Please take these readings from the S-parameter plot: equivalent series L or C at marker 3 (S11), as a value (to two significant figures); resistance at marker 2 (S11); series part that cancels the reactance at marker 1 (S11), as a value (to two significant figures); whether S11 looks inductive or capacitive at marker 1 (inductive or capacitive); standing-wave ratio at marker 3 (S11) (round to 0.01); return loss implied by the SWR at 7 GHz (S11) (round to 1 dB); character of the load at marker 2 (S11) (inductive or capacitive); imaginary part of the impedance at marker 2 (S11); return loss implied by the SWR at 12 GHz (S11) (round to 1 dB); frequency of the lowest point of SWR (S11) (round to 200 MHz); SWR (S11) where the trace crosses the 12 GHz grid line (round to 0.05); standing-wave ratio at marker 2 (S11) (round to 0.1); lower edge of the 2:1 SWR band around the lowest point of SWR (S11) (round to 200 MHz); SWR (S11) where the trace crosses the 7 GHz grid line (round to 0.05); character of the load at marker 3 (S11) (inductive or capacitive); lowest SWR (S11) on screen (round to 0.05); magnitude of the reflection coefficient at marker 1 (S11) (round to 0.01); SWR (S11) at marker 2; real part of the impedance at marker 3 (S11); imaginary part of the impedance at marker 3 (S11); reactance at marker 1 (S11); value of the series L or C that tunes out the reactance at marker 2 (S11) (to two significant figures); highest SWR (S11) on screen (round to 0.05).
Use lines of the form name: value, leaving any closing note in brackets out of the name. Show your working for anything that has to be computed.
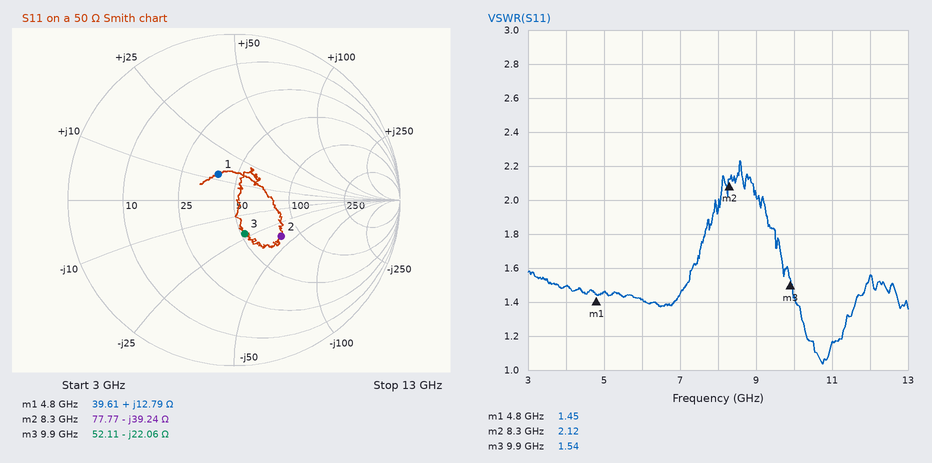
equivalent series L or C at marker 3 (S11), as a value: C = 1/(2π × 9.9 GHz × 22.06 Ω) ≈ 729 fF, so 730 fF to two significant figures
resistance at marker 2: 77.77 Ω
series part that cancels the reactance at marker 1 (S11), as a value: C = 1/(2π × 4.8 GHz × 12.79 Ω) ≈ 2.6 pF
whether S11 looks inductive or capacitive at marker 1: inductive
standing-wave ratio at marker 3 (S11): 1.54
return loss implied by the SWR at 7 GHz (S11): −20 log10((1.45 − 1)/(1.45 + 1)) ≈ 15 dB
character of the load at marker 2 (S11): capacitive
imaginary part of the impedance at marker 2: -39.24 Ω
return loss implied by the SWR at 12 GHz (S11): −20 log10((1.55 − 1)/(1.55 + 1)) ≈ 13 dB
frequency of the lowest point of SWR (S11): 10.8 GHz
SWR (S11) where the trace crosses the 12 GHz grid line: 1.55
standing-wave ratio at marker 2 (S11): 2.1
lower edge of the 2:1 SWR band around the lowest point of SWR (S11): 9.2 GHz
SWR (S11) where the trace crosses the 7 GHz grid line: 1.45
character of the load at marker 3 (S11): capacitive
lowest SWR (S11) on screen: 1.05
magnitude of the reflection coefficient at marker 1 (S11): 0.18
SWR (S11) at marker 2: 2.12
real part of the impedance at marker 3: 52.11 Ω
imaginary part of the impedance at marker 3: -22.06 Ω
reactance at marker 1: +12.79 Ω
value of the series L or C that tunes out the reactance at marker 2 (S11): L = 39.24 Ω/(2π × 8.3 GHz) ≈ 752 pH, so 750 pH to two significant figures
highest SWR (S11) on screen: 2.25
